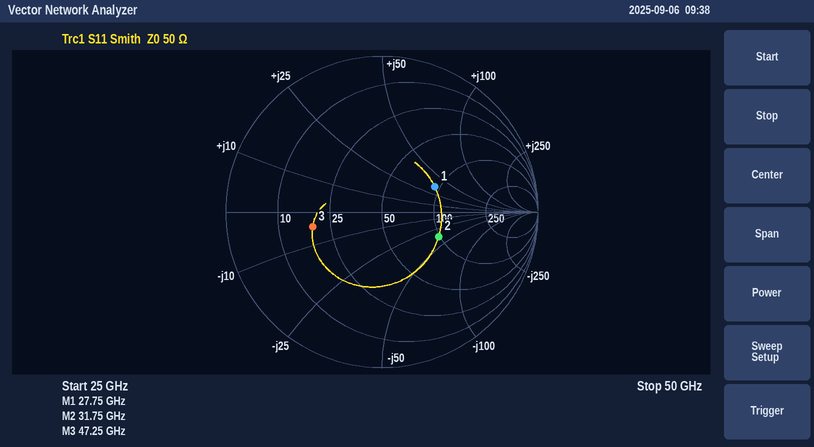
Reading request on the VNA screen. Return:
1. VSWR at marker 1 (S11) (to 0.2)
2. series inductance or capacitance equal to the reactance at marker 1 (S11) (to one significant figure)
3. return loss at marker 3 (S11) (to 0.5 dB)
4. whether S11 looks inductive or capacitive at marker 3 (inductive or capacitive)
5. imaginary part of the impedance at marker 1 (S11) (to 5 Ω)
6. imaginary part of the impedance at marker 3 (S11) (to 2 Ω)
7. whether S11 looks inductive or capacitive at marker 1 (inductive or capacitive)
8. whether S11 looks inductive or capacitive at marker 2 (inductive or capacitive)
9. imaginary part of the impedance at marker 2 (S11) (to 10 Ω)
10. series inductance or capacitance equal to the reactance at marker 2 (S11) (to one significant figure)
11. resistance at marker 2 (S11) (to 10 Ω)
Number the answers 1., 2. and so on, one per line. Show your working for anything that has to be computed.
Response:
1. 2.2
2. L = 35 Ω/(2π × 27.75 GHz) ≈ 201 pH, so 200 pH to one significant figure
3. 7.0 dB
4. capacitive
5. +35 Ω
6. -4 Ω
7. inductive
8. capacitive
9. -40 Ω
10. C = 1/(2π × 31.75 GHz × 40 Ω) ≈ 125 fF, so 100 fF to one significant figure
11. 100 Ω
